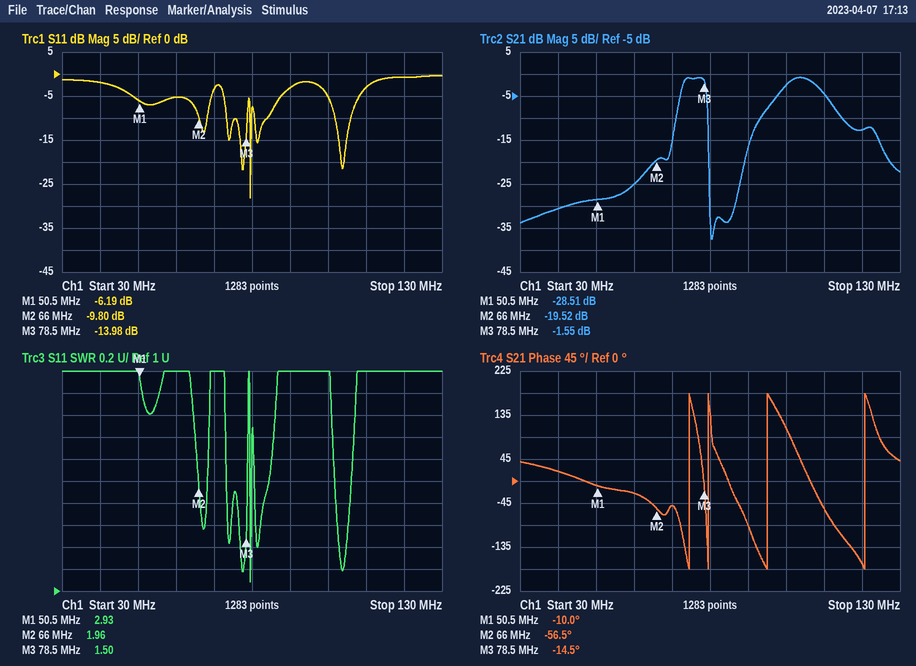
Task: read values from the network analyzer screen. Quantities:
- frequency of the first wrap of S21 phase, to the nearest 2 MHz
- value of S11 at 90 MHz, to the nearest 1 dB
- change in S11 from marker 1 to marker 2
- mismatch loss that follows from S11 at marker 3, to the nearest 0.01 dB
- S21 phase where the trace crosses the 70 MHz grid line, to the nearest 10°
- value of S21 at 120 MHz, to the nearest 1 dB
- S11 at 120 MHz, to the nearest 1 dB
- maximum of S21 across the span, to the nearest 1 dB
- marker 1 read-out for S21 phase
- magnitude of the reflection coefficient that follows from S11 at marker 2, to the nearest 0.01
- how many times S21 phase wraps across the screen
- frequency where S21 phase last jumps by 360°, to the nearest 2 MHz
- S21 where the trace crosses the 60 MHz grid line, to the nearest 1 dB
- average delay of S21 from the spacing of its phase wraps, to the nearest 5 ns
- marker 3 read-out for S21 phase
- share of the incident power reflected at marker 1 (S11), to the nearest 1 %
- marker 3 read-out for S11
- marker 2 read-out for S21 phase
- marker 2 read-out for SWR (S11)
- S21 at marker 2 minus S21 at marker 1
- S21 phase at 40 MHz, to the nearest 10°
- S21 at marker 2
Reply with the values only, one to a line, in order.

74 MHz
-3 dB
-3.61 dB
0.18 dB
-50°
-13 dB
-1 dB
-1 dB
-10.0°
0.32
4
120 MHz
-25 dB
65 ns
-14.5°
24 %
-13.98 dB
-56.5°
1.96
8.99 dB
20°
-19.52 dB
